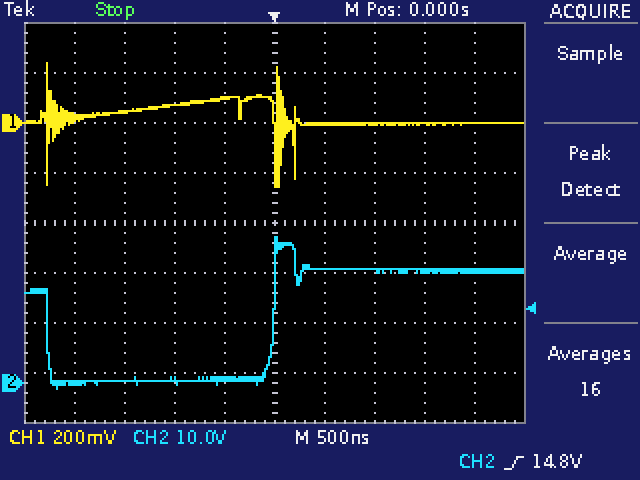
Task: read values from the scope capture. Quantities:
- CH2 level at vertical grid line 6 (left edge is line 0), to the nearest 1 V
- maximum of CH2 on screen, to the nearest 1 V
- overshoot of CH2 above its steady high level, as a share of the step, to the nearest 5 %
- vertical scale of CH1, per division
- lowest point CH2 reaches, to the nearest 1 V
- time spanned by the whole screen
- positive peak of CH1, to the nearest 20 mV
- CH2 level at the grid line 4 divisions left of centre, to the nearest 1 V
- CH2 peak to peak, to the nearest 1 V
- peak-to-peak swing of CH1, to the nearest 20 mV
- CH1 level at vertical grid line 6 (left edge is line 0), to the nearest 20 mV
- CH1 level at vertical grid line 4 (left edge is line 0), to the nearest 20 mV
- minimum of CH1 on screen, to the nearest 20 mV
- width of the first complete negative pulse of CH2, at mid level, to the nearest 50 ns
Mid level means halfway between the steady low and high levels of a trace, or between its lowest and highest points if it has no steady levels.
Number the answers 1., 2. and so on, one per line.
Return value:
1. 23 V
2. 29 V
3. 30 %
4. 200 mV
5. -1 V
6. 5 µs
7. 240 mV
8. 0 V
9. 30 V
10. 500 mV
11. 0 mV
12. 100 mV
13. -260 mV
14. 2.25 µs
